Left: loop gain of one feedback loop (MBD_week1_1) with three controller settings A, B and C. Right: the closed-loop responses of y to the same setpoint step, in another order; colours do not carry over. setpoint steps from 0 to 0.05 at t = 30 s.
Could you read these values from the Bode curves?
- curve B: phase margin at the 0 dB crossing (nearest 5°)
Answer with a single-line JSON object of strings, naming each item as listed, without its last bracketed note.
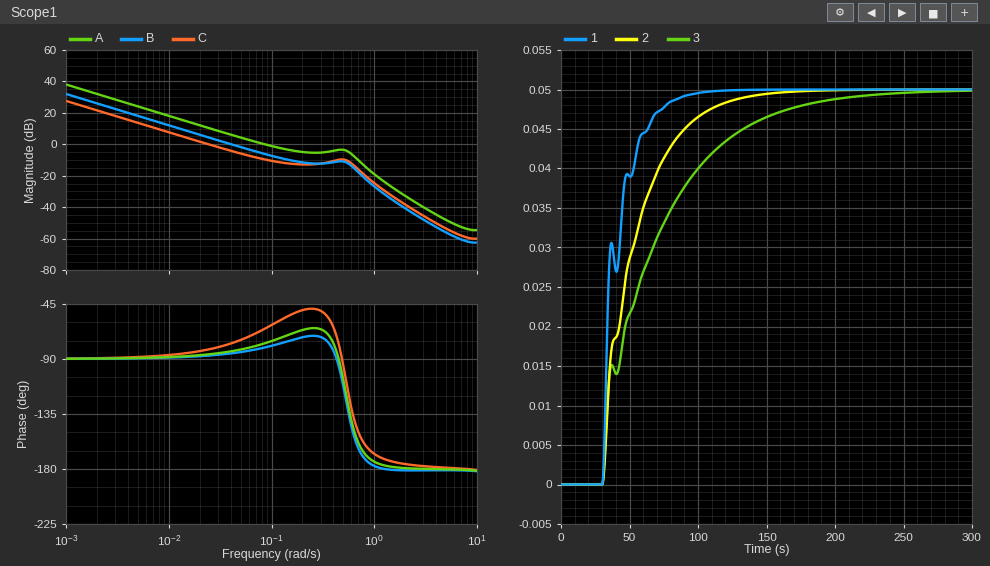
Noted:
{"curve B: phase margin at the 0 dB crossing": "95°"}
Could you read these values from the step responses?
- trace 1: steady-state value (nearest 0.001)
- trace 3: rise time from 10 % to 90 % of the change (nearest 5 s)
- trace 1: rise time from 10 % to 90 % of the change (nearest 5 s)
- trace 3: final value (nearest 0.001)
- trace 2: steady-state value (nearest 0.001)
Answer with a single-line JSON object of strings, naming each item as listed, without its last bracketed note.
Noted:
{"trace 1: steady-state value": "0.050", "trace 3: rise time from 10 % to 90 % of the change": "100 s", "trace 1: rise time from 10 % to 90 % of the change": "30 s", "trace 3: final value": "0.050", "trace 2: steady-state value": "0.050"}
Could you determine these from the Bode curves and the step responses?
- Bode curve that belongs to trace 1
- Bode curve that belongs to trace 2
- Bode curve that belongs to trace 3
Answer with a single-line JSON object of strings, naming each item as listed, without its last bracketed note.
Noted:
{"Bode curve that belongs to trace 1": "A", "Bode curve that belongs to trace 2": "B", "Bode curve that belongs to trace 3": "C"}
